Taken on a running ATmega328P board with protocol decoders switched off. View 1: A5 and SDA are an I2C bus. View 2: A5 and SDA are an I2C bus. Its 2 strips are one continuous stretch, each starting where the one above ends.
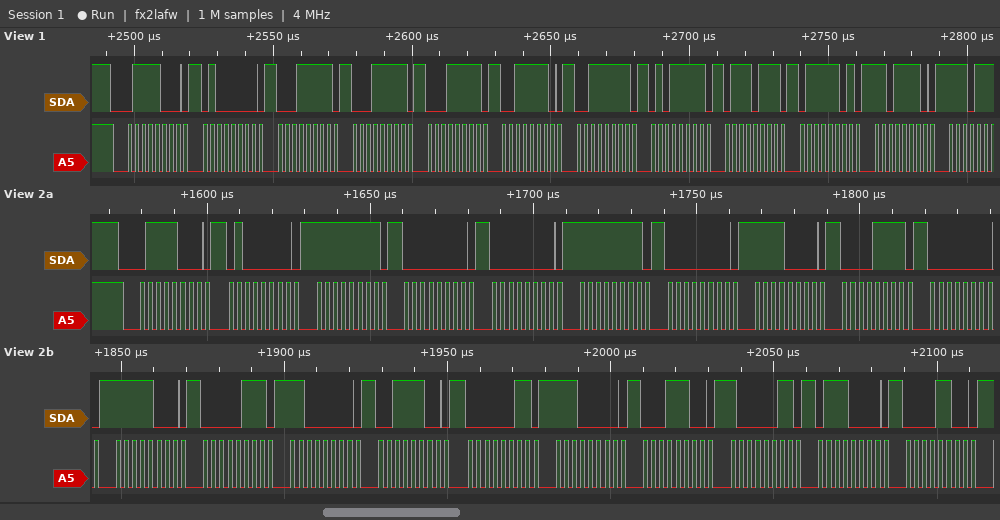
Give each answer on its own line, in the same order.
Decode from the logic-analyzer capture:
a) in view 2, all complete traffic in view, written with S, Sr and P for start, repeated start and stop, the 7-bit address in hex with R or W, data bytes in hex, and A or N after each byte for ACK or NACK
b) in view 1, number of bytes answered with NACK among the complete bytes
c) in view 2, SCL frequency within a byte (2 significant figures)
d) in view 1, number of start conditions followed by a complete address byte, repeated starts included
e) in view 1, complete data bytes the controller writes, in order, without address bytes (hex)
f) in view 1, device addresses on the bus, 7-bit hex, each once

S 3CW A 40 A FF A 00 A 00 A FF A 00 A F0 A 0F A 00 A F8 A 07 A C0 A 3C A 03 A E0 A 1C A 83 A 70 A 0C A
0
400 kHz
1
40 1F 1F 1F 3E 3F 5F 77 7D DE
0x3C
